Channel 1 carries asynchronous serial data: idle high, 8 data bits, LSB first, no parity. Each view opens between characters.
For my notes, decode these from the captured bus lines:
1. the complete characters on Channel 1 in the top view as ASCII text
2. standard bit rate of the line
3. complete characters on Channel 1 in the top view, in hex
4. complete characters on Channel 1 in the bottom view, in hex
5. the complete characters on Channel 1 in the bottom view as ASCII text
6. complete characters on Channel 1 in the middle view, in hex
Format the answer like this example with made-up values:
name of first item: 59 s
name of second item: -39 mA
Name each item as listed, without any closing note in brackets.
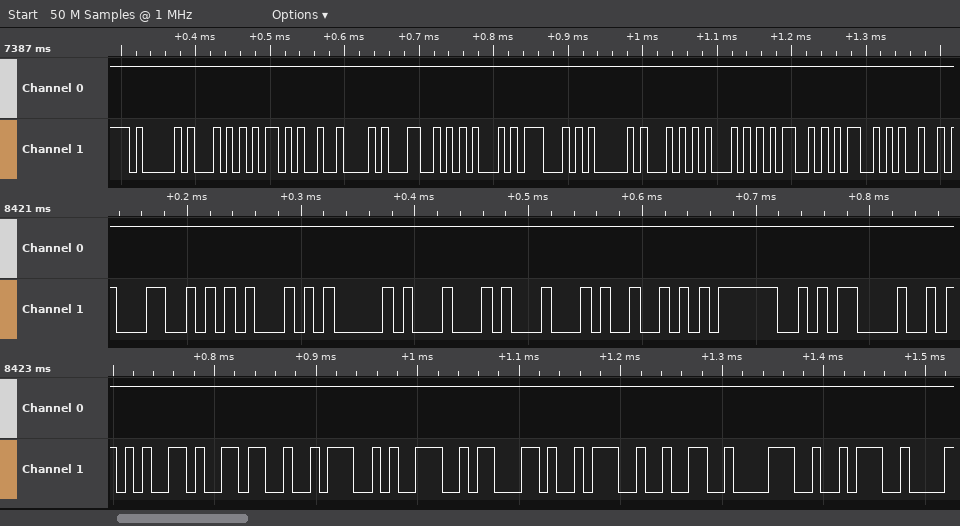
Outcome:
the complete characters on Channel 1 in the top view as ASCII text: "AT+BLEGATTSS"
standard bit rate of the line: 115200 baud
complete characters on Channel 1 in the top view, in hex: 41, 54, 2B, 42, 4C, 45, 47, 41, 54, 54, 53, 53
complete characters on Channel 1 in the bottom view, in hex: 65, 36, 3A, 39, 63, 3A, 32, 38, 3A
the complete characters on Channel 1 in the bottom view as ASCII text: "e6:9c:28:"
complete characters on Channel 1 in the middle view, in hex: 4C, 45, 41, 44, 44, 52, 3F, 0D
